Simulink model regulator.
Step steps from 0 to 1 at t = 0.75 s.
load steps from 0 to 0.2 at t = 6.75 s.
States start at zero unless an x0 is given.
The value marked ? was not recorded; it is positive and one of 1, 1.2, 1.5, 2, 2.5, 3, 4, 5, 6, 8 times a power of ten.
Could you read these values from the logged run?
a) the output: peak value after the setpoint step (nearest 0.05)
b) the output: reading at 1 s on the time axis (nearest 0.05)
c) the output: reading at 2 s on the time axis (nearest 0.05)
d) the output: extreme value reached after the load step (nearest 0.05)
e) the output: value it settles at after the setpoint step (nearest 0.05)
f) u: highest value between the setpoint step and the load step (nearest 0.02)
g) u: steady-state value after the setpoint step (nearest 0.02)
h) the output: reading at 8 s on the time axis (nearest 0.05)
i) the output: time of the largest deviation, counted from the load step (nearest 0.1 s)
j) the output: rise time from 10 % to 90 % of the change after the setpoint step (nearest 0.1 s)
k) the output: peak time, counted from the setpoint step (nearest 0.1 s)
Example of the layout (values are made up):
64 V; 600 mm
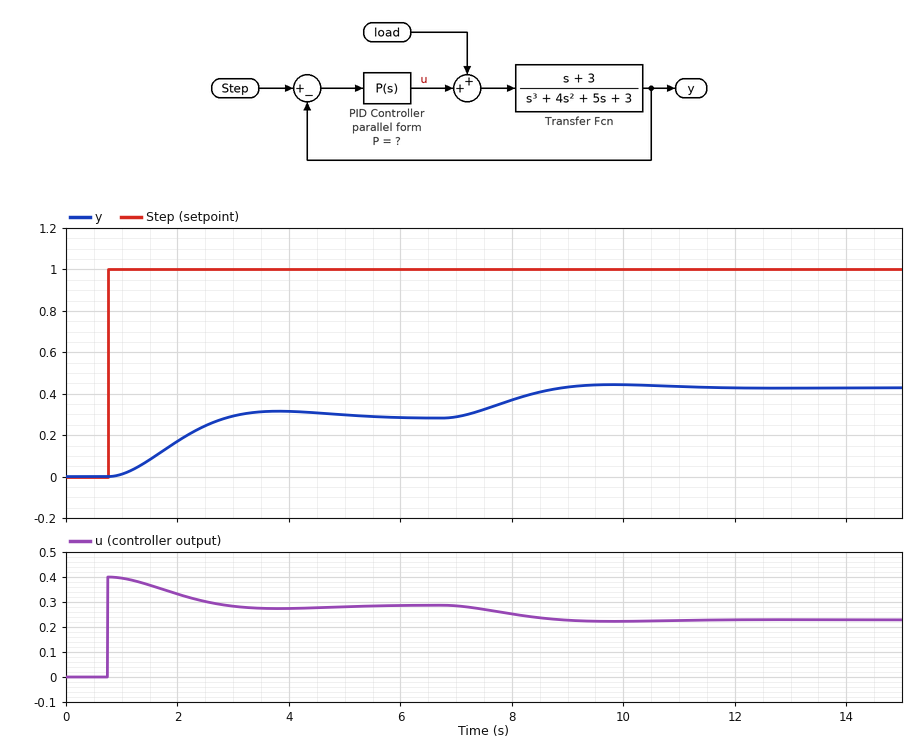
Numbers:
0.30; 0.00; 0.15; 0.45; 0.30; 0.40; 0.28; 0.35; 3.1 s; 1.4 s; 3.1 s
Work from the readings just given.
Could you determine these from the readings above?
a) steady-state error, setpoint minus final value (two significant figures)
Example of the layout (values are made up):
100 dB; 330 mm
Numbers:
0.70
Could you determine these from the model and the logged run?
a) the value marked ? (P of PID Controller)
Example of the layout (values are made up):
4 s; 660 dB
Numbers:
0.4
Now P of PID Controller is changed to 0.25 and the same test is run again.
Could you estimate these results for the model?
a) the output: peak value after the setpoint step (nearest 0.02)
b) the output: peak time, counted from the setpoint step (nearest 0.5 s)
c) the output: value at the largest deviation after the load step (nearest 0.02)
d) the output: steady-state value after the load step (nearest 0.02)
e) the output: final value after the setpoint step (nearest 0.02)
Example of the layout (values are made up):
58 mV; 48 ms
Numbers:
0.22; 3.5 s; 0.38; 0.36; 0.20
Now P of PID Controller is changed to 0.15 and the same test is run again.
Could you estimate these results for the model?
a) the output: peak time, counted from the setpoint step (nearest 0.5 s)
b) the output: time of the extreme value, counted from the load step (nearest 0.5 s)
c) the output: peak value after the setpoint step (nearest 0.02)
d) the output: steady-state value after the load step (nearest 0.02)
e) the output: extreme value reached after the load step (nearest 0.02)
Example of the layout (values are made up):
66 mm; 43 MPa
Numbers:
3.5 s; 3.5 s; 0.14; 0.30; 0.32
